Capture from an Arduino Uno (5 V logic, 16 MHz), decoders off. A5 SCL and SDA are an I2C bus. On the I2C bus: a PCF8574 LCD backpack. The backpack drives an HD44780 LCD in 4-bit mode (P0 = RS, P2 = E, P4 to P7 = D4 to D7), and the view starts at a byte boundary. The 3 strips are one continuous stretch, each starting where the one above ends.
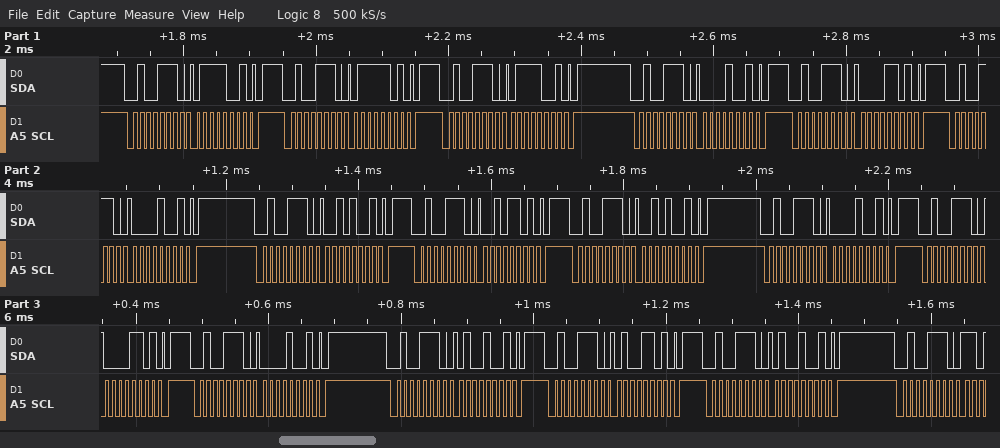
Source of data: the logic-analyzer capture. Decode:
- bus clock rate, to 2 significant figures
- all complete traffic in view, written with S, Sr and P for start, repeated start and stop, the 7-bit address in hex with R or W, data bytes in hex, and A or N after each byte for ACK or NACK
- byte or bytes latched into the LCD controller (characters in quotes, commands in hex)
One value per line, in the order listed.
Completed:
100 kHz
S 27W A 79 A P S 27W A 7D A P S 27W A 79 A P S 27W A 09 A P S 27W A 0D A P S 27W A 09 A P S 27W A 29 A P S 27W A 2D A P S 27W A 29 A P S 27W A 09 A P S 27W A 0D A P S 27W A 09 A P S 27W A 49 A P S 27W A 4D A P S 27W A 49 A P S 27W A
'p' ' '
